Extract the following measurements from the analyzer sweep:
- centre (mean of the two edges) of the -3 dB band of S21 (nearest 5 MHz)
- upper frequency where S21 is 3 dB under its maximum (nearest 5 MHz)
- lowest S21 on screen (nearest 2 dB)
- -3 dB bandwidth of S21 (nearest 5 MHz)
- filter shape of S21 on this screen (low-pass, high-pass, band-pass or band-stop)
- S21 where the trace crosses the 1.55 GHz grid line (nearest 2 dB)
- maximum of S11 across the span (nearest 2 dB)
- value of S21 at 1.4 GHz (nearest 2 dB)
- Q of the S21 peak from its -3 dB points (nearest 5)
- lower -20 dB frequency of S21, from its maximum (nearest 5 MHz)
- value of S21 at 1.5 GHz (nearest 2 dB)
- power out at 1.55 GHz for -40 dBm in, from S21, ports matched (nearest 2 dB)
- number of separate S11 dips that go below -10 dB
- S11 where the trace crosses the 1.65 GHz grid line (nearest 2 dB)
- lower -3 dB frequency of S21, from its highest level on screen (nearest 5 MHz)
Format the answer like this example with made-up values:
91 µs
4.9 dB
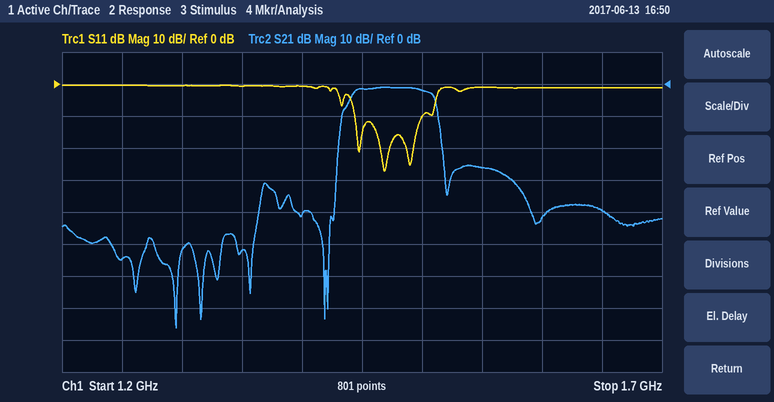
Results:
1.475 GHz
1.510 GHz
-76 dB
70 MHz
band-pass
-26 dB
0 dB
-40 dB
20
1.430 GHz
-2 dB
-66 dBm
3
-2 dB
1.440 GHz
